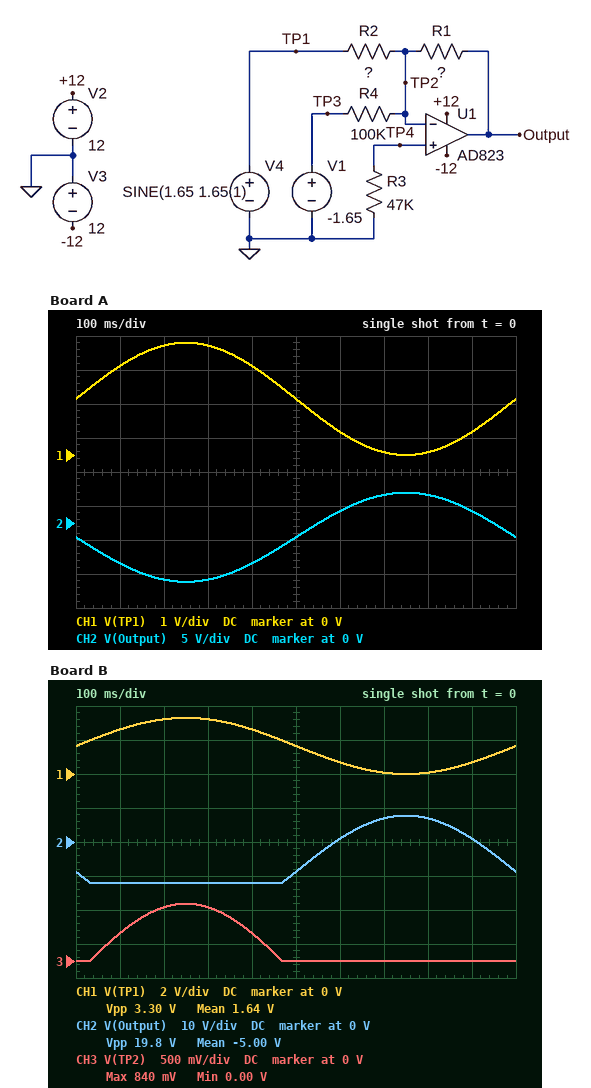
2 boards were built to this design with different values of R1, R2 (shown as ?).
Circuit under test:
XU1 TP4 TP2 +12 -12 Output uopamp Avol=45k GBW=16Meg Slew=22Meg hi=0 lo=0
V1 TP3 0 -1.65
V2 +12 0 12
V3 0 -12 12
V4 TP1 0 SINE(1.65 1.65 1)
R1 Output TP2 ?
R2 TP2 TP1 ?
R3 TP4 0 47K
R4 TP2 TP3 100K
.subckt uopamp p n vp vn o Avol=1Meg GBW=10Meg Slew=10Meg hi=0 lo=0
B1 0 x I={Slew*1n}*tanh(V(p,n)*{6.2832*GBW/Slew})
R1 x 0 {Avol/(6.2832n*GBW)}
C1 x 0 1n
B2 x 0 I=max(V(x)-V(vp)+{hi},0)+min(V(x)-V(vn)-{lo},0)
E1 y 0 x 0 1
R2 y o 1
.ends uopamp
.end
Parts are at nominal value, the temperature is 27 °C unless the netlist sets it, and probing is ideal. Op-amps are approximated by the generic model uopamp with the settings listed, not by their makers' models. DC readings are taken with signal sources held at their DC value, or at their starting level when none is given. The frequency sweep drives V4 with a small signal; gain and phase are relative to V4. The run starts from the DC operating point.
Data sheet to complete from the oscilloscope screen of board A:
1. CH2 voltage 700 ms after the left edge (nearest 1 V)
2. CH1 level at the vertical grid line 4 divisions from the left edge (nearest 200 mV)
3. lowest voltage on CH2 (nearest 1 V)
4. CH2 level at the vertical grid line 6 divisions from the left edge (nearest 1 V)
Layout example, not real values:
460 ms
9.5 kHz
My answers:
4 V
2.6 V
-9 V
2 V
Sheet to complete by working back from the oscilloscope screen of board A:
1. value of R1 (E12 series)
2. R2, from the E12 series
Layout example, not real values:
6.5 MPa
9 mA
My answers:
270 kΩ
68 kΩ
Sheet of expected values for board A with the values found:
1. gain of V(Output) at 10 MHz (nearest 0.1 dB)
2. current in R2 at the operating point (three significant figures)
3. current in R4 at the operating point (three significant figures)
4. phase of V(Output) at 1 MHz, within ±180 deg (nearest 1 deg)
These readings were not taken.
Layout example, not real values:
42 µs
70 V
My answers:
-1.8 dB
24.3 µA
16.5 µA
154 deg
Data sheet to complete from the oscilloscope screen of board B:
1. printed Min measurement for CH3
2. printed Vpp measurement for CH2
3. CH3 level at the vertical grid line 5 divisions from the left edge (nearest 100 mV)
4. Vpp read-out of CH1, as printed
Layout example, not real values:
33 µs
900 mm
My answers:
0.00 V
19.8 V
0 V
3.30 V
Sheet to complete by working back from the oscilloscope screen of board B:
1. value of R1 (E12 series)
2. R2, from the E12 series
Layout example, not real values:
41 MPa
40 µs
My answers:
470 kΩ
47 kΩ
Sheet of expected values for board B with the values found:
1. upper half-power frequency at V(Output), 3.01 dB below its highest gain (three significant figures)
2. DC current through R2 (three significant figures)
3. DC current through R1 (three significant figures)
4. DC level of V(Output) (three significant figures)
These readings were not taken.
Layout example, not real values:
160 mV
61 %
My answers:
1.02 MHz
35.1 µA
18.6 µA
-8.74 V
